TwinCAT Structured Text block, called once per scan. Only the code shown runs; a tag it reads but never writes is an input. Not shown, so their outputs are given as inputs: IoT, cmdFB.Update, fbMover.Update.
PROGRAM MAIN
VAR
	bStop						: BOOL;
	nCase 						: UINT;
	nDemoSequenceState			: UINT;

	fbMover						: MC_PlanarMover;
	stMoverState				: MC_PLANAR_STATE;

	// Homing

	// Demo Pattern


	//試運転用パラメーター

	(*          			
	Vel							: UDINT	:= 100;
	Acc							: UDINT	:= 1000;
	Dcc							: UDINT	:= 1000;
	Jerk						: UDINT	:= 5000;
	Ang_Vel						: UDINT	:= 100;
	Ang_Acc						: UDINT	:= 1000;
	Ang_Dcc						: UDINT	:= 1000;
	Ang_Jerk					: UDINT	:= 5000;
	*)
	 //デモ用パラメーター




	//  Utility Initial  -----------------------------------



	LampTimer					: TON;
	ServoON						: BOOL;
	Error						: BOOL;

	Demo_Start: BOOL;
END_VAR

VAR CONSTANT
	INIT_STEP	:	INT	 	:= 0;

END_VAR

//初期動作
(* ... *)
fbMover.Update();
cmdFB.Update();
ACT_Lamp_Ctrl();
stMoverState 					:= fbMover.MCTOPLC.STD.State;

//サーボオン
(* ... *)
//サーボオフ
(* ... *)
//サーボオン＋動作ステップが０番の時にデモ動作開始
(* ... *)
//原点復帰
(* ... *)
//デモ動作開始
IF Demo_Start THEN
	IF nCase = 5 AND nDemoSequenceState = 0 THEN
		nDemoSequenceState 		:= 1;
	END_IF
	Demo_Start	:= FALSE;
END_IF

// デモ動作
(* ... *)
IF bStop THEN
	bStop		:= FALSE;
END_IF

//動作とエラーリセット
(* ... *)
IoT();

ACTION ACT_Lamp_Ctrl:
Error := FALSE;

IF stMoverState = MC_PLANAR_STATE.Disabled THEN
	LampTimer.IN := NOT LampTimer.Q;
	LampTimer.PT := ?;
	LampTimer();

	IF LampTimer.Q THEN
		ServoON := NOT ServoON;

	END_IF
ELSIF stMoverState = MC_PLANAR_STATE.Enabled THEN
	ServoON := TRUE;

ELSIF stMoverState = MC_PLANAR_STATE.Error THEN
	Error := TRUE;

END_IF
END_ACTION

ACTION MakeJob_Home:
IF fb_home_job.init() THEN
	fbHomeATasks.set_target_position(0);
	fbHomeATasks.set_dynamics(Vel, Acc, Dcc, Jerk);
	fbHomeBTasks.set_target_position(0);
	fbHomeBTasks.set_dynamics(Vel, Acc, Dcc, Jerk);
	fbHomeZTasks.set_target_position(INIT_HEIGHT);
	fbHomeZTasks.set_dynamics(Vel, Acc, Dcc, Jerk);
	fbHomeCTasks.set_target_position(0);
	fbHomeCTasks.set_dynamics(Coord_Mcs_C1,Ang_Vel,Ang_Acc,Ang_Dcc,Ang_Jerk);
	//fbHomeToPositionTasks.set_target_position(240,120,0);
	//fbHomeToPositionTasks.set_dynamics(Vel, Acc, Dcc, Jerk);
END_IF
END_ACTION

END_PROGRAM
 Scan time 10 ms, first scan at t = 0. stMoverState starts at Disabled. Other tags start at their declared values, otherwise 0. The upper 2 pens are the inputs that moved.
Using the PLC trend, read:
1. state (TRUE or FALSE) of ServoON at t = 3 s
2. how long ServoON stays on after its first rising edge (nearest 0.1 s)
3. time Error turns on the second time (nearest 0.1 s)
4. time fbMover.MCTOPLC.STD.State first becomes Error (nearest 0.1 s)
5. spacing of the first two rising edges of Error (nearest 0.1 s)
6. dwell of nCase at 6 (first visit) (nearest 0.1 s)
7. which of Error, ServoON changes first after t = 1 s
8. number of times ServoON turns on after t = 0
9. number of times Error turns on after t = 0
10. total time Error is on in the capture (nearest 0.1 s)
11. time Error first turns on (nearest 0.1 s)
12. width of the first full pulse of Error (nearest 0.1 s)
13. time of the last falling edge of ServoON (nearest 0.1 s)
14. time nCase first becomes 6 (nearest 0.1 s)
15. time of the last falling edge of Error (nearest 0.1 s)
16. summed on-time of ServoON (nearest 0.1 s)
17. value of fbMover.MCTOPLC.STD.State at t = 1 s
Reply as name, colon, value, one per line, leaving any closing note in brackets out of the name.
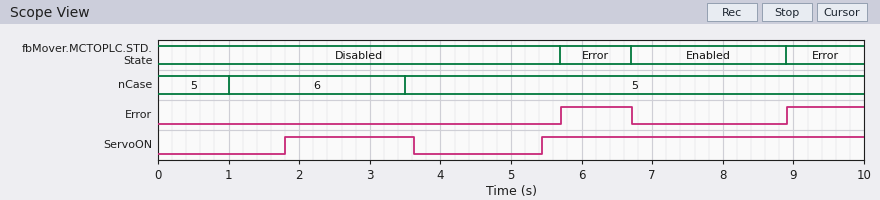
state (TRUE or FALSE) of ServoON at t = 3 s: TRUE
how long ServoON stays on after its first rising edge: 1.8 s
time Error turns on the second time: 8.9 s
time fbMover.MCTOPLC.STD.State first becomes Error: 5.7 s
spacing of the first two rising edges of Error: 3.2 s
dwell of nCase at 6 (first visit): 2.5 s
which of Error, ServoON changes first after t = 1 s: ServoON
number of times ServoON turns on after t = 0: 2
number of times Error turns on after t = 0: 2
total time Error is on in the capture: 2.1 s
time Error first turns on: 5.7 s
width of the first full pulse of Error: 1.0 s
time of the last falling edge of ServoON: 3.6 s
time nCase first becomes 6: 1.0 s
time of the last falling edge of Error: 6.7 s
summed on-time of ServoON: 6.4 s
value of fbMover.MCTOPLC.STD.State at t = 1 s: Disabled
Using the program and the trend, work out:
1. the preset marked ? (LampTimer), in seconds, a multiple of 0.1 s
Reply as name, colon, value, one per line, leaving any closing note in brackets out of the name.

the preset marked ? (LampTimer), in seconds, a multiple of 0.1 s: 1.8 s
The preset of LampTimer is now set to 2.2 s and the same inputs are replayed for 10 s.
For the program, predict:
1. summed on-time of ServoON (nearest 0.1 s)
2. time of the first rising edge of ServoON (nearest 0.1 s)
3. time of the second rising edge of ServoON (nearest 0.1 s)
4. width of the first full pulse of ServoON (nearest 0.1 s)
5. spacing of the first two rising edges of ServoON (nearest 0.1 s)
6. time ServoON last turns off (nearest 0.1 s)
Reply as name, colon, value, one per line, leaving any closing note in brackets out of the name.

summed on-time of ServoON: 5.5 s
time of the first rising edge of ServoON: 2.2 s
time of the second rising edge of ServoON: 6.7 s
width of the first full pulse of ServoON: 2.2 s
spacing of the first two rising edges of ServoON: 4.5 s
time ServoON last turns off: 4.4 s
